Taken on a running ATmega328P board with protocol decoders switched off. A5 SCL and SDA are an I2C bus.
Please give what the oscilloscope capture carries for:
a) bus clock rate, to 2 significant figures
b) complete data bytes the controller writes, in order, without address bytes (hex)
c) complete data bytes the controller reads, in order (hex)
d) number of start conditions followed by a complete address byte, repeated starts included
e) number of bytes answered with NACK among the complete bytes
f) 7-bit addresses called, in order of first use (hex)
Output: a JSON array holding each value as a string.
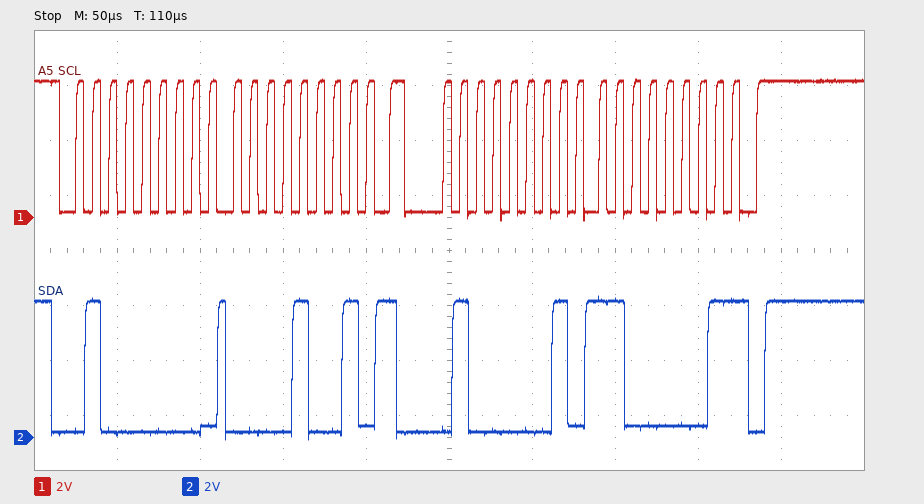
["100 kHz", "09", "C1", "2", "1", "0x20"]
